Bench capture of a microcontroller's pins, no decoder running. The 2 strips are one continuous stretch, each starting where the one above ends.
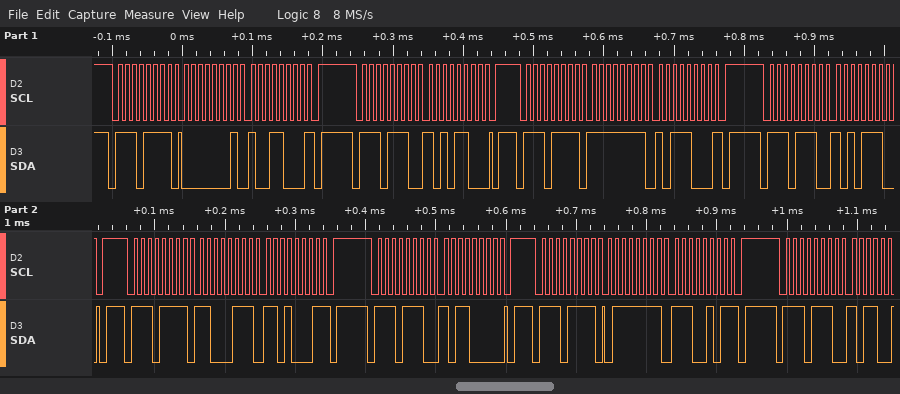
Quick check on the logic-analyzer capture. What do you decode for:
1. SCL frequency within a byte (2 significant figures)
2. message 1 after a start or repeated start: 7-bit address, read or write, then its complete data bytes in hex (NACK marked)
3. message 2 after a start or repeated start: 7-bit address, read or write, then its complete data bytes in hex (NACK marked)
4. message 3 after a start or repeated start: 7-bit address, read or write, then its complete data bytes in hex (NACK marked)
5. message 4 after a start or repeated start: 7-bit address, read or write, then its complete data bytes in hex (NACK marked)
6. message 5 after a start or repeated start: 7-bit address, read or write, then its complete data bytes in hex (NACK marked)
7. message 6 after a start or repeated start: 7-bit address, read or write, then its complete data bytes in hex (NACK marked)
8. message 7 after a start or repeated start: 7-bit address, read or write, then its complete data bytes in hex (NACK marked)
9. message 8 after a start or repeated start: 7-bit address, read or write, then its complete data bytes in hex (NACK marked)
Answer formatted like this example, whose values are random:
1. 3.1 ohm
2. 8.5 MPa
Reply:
1. 100 kHz
2. 0x77 read: 01 98 NACK
3. 0x77 write: AC
4. 0x77 read: FF B8 NACK
5. 0x77 write: AE
6. 0x77 read: C7 D1 NACK
7. 0x77 write: B0
8. 0x77 read: 7F E5 NACK
9. 0x77 write
